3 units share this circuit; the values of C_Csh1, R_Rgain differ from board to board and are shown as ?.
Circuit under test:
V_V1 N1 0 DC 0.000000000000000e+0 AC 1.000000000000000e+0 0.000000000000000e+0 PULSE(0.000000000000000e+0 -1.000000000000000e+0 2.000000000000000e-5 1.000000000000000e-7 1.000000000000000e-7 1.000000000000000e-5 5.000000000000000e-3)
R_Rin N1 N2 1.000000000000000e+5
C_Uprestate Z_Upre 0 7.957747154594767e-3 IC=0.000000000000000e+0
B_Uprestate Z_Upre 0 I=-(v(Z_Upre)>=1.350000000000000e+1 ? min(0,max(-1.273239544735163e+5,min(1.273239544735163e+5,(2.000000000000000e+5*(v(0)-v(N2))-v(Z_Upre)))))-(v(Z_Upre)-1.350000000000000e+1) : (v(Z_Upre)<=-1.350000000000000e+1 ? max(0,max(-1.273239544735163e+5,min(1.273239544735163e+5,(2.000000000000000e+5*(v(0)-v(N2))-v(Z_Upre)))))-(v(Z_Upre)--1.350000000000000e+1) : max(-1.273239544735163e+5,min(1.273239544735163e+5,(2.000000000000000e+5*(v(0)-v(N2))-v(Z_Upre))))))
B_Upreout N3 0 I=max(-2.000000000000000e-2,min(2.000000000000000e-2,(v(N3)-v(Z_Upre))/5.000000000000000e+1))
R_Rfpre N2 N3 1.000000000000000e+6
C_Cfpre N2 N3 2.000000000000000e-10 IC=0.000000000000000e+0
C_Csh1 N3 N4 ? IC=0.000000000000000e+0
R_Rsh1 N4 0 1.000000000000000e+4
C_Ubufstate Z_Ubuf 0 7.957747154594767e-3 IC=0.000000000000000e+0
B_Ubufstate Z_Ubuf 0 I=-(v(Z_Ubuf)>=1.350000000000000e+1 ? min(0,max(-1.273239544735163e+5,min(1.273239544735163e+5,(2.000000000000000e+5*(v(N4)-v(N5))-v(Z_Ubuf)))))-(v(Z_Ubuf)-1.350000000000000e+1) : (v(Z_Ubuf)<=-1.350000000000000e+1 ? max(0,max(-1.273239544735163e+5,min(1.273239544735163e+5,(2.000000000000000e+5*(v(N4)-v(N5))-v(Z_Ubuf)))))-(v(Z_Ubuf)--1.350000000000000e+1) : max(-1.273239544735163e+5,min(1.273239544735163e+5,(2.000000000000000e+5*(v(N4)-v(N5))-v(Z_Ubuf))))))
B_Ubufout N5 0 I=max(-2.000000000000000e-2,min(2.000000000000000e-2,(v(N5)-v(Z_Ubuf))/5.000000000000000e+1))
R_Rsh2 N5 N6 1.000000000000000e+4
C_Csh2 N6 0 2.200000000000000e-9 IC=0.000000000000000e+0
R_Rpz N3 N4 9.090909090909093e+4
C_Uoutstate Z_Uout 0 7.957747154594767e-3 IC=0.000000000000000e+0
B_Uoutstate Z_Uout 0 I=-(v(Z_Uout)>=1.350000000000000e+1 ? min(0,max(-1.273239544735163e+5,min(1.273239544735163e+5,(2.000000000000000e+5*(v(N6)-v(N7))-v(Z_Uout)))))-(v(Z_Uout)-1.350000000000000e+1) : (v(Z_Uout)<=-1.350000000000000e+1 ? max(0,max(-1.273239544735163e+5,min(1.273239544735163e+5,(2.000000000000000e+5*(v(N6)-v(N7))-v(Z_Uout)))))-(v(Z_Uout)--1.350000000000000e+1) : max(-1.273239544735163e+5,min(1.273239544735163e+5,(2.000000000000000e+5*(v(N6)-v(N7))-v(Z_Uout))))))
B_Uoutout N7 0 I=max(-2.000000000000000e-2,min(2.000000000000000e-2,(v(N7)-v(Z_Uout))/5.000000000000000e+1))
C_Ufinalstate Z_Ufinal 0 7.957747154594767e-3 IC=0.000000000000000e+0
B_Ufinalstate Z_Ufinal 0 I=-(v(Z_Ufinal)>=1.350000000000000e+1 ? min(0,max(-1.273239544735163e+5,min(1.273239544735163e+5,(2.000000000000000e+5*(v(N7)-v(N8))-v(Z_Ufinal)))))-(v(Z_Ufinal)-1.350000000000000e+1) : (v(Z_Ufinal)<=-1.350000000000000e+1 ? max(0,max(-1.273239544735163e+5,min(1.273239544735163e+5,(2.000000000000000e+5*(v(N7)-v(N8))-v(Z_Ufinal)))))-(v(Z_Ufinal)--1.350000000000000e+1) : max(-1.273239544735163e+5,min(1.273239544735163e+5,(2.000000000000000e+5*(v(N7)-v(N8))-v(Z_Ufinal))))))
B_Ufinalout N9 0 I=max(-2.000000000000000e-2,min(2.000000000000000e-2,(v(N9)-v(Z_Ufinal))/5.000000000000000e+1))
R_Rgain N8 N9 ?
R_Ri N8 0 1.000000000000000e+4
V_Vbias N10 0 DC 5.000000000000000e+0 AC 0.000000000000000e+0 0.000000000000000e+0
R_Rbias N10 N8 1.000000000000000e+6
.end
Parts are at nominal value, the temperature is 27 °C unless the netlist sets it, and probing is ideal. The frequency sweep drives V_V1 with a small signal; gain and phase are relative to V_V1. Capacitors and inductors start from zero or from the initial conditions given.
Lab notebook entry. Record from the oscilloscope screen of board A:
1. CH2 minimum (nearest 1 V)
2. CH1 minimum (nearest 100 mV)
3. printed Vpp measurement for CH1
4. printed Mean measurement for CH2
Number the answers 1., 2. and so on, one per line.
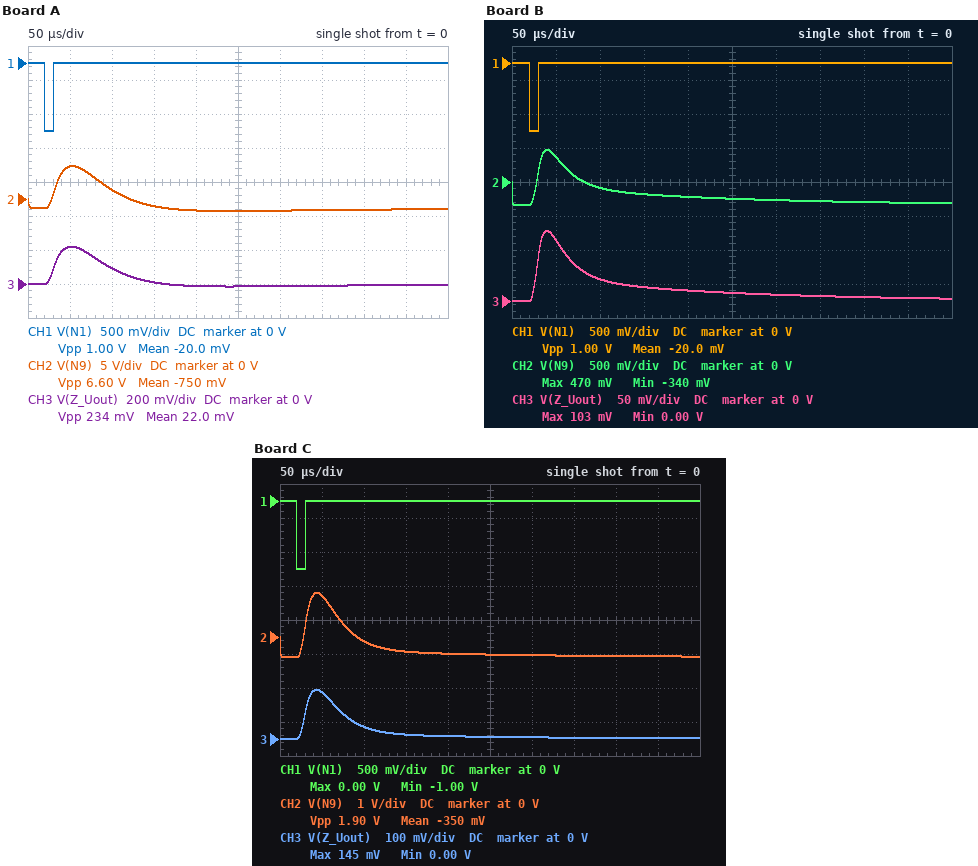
1. -2 V
2. -1.0 V
3. 1.00 V
4. -750 mV
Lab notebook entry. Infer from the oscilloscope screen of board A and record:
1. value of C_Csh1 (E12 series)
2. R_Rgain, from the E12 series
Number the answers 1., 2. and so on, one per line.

1. 3.9 nF
2. 270 kΩ
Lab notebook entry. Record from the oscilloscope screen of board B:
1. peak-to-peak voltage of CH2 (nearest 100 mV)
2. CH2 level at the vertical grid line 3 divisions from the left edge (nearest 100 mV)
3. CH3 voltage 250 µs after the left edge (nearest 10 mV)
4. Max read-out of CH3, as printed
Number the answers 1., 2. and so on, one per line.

1. 800 mV
2. -200 mV
3. 10 mV
4. 103 mV
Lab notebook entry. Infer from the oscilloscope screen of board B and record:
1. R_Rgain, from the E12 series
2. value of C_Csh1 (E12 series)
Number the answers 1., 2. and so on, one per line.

1. 68 kΩ
2. 820 pF
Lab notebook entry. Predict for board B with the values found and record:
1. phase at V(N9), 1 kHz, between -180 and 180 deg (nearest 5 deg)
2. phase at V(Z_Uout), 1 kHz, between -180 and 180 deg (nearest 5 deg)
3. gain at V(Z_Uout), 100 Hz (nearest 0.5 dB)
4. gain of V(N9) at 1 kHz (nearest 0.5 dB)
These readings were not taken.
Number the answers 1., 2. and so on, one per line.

1. 145 deg
2. 145 deg
3. 0 dB
4. 14.5 dB
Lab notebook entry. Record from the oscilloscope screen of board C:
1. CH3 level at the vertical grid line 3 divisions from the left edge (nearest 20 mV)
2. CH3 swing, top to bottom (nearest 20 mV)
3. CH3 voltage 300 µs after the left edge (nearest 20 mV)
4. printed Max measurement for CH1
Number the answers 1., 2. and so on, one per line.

1. 20 mV
2. 140 mV
3. 0 V
4. 0.00 V
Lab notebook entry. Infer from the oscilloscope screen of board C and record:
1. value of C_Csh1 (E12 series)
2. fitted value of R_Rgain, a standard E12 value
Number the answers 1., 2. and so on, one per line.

1. 1.5 nF
2. 120 kΩ
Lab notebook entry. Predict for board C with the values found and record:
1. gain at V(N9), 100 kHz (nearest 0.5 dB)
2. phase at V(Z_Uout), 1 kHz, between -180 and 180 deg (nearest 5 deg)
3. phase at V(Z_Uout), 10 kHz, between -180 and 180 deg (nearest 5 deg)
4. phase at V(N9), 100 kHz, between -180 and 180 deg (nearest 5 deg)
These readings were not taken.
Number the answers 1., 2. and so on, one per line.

1. -23.0 dB
2. 155 deg
3. 85 deg
4. -10 deg
